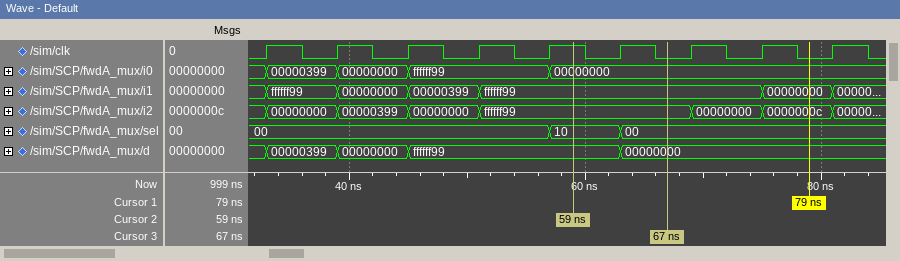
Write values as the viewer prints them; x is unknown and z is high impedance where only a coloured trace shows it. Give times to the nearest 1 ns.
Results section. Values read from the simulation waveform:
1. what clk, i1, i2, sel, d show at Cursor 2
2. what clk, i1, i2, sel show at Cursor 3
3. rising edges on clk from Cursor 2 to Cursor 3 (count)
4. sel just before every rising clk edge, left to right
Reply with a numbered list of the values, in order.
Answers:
1. clk=1, i1=ffffff99, i2=ffffff99, sel=10, d=ffffff99
2. clk=0, i1=ffffff99, i2=ffffff99, sel=00
3. 1
4. 00, 00, 00, 00, 00, 10, 00, 00, 00
